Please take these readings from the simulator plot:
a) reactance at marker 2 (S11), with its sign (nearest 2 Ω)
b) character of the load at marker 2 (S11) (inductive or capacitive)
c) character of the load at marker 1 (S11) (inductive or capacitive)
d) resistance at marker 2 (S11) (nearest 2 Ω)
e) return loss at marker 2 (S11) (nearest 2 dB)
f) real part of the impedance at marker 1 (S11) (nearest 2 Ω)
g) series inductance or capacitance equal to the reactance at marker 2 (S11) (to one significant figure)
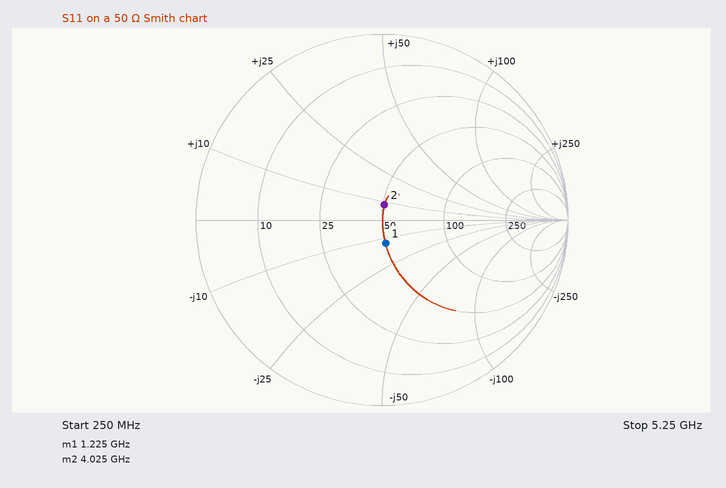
+8 Ω
inductive
capacitive
50 Ω
22 dB
50 Ω
300 pH
